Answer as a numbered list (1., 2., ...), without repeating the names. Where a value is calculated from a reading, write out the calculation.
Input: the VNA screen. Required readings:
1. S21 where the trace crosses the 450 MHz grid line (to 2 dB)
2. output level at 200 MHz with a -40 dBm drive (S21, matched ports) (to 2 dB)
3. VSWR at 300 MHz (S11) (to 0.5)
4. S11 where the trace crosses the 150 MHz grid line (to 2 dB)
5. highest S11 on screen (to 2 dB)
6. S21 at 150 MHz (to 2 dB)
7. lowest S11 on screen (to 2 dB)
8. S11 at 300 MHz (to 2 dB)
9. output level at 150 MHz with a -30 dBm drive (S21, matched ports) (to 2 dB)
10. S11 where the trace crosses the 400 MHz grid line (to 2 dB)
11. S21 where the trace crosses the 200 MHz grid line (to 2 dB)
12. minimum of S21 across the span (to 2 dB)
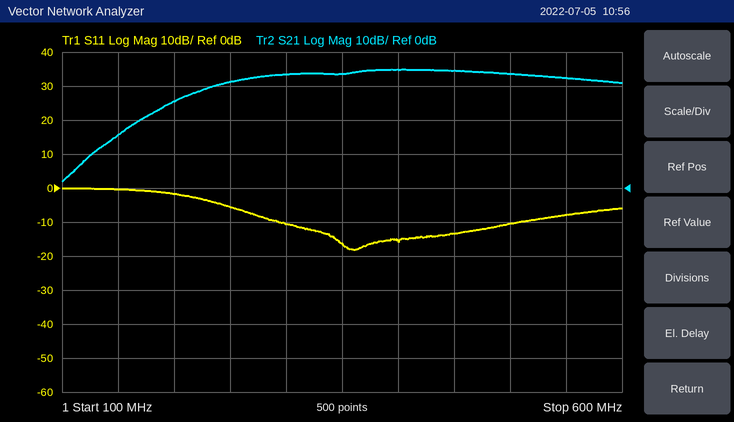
1. 34 dB
2. -40 dBm + (26 dB) = -14 dBm
3. |Γ| = 10^(-10/20) = 0.3162; VSWR = (1 + 0.3162)/(1 − 0.3162) ≈ 1.92, so 2.0 to the nearest 0.5
4. 0 dB
5. 0 dB
6. 16 dB
7. -18 dB
8. -10 dB
9. -30 dBm + (16 dB) = -14 dBm
10. -16 dB
11. 26 dB
12. 2 dB
